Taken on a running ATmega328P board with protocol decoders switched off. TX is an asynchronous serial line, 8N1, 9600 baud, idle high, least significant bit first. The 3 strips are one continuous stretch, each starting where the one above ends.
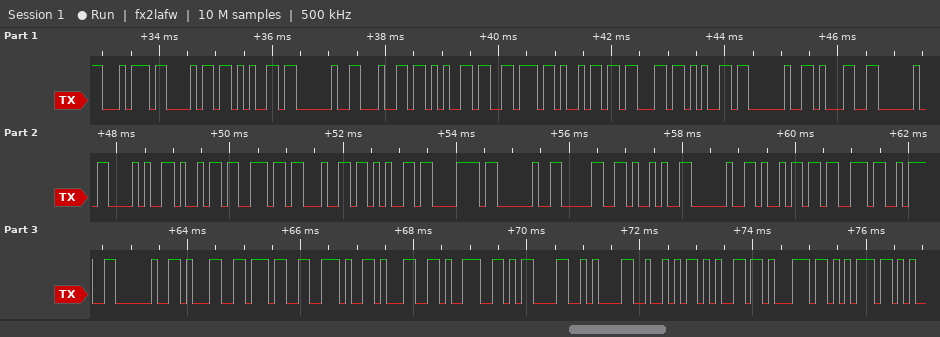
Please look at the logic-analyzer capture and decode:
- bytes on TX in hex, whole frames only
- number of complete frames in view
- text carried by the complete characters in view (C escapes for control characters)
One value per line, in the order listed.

74 68 65 20 64 65 76 69 63 65 20 31 20 28 69 6E 64 65 78 20 30 29 20 69 73 3A 20 31 37 2E 31 39 0D 0A 52 65 71 75
38
"the device 1 (index 0) is: 17.19\r\nRequ"
